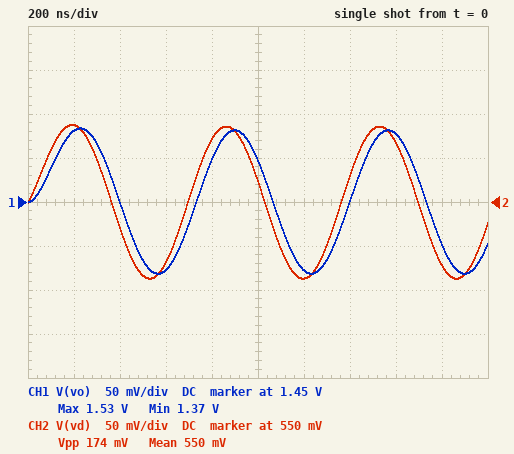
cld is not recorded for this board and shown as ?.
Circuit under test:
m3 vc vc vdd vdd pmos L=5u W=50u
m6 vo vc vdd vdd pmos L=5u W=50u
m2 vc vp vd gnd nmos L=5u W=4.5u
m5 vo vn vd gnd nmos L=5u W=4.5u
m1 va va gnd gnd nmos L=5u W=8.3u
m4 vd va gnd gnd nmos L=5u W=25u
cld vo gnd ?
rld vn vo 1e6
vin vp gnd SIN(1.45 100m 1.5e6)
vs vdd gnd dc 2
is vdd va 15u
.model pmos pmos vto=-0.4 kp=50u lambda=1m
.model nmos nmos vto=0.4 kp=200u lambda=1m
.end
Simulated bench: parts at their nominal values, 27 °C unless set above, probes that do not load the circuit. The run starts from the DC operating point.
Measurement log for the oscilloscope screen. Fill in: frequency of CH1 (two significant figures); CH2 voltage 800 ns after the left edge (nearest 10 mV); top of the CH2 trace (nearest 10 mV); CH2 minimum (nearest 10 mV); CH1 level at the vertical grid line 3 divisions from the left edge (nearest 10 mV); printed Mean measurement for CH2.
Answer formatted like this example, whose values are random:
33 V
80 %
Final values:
1.5 MHz
620 mV
640 mV
460 mV
1.37 V
550 mV
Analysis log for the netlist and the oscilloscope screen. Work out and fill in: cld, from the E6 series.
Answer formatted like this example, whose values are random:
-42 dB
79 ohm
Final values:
6.8 pF
